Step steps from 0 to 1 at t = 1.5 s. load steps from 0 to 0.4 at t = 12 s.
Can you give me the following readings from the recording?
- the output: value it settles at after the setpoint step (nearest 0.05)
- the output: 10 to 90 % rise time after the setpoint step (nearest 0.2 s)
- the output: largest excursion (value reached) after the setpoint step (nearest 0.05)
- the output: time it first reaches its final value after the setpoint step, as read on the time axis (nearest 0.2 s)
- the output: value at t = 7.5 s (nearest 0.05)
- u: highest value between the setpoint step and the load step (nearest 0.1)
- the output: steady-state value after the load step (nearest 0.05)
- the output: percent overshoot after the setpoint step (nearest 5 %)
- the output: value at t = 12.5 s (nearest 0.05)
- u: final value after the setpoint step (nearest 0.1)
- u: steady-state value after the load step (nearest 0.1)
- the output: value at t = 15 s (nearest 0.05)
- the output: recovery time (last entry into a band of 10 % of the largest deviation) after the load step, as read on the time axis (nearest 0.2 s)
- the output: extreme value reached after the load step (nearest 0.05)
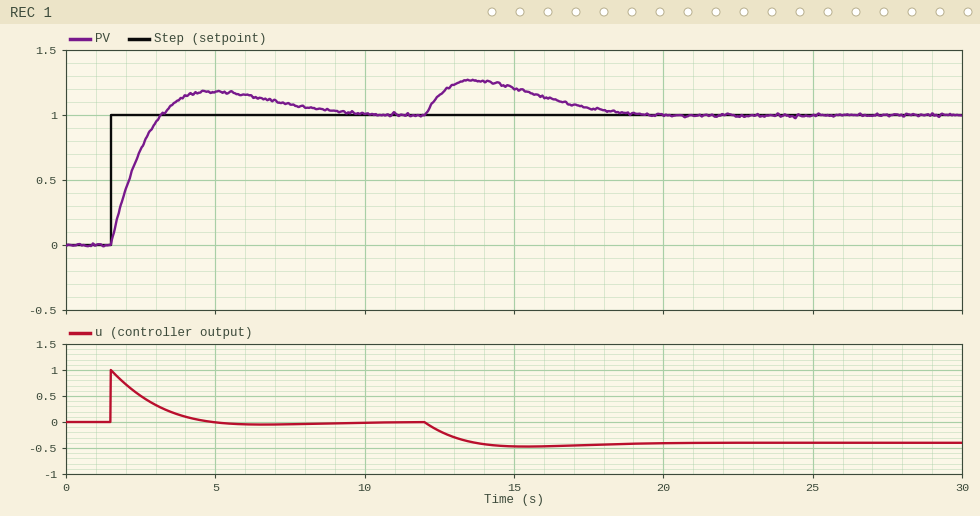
1.00
1.2 s
1.20
3.2 s
1.10
1.0
1.00
20 %
1.15
0.0
-0.4
1.20
18.4 s
1.25
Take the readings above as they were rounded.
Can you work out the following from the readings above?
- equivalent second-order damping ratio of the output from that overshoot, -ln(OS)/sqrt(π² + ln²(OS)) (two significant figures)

0.46
